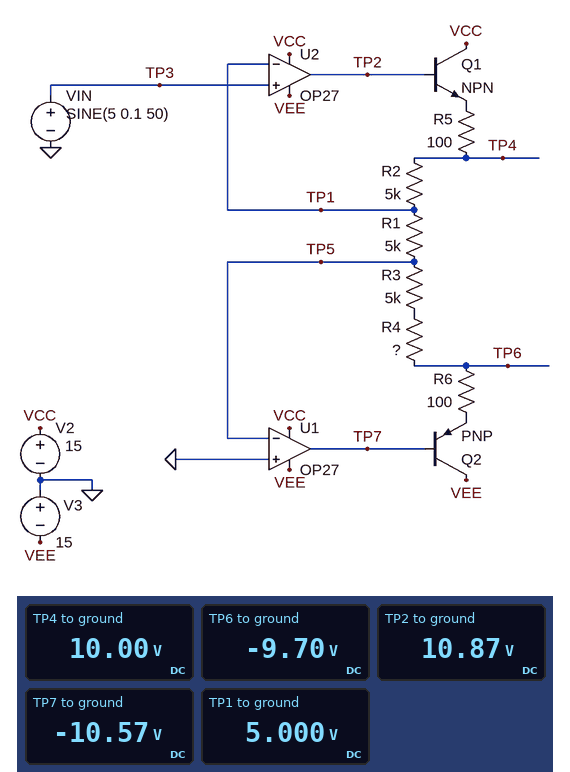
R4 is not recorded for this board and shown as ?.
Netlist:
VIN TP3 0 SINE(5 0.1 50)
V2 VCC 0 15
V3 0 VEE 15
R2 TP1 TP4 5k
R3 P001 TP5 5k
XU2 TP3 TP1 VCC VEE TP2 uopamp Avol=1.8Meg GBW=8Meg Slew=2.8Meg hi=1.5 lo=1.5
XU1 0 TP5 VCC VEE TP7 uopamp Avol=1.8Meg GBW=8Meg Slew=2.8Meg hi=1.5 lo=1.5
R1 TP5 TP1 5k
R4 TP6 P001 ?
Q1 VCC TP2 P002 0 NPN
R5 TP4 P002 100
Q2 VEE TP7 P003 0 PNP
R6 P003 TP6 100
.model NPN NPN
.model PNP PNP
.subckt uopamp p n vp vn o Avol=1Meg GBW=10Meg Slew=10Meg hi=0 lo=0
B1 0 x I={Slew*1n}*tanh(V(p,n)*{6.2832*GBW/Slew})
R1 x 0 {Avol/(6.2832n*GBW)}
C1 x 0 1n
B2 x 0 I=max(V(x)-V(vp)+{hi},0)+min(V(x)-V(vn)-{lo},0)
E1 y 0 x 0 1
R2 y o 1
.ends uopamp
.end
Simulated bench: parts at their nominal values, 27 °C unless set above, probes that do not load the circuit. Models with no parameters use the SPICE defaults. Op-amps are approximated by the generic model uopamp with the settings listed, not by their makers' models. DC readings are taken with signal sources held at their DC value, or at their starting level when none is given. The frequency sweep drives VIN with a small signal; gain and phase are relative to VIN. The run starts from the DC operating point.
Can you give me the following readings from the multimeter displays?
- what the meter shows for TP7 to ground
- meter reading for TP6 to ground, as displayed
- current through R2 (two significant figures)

-10.57 V
-9.70 V
1.0 mA
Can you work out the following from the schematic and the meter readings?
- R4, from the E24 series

4.7 kΩ
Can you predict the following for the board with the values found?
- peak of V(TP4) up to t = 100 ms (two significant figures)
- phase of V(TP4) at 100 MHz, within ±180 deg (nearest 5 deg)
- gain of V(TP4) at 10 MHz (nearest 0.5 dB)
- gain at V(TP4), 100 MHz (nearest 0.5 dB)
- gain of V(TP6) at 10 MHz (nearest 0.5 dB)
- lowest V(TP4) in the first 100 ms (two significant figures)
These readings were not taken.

10 V
-85 deg
-3.5 dB
-22.0 dB
-12.5 dB
9.8 V
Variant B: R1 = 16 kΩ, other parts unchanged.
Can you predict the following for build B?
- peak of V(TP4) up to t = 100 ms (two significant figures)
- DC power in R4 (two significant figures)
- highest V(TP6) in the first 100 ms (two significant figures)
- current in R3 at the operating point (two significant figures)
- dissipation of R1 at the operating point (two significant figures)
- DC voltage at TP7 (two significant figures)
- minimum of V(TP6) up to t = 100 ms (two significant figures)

6.7 V
460 µW
-3.0 V
310 µA
1.6 mW
-3.8 V
-3.1 V
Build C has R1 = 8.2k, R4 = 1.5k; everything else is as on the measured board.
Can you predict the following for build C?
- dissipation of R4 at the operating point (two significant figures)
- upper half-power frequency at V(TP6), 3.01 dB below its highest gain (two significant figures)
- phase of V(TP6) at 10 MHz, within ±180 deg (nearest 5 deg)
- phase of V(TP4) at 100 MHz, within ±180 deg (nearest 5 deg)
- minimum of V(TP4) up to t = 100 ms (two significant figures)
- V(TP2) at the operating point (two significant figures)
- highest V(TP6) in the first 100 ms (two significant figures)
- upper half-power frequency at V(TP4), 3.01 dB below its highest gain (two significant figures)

560 µW
2.9 MHz
55 deg
-85 deg
7.9 V
8.9 V
-3.9 V
4.0 MHz
